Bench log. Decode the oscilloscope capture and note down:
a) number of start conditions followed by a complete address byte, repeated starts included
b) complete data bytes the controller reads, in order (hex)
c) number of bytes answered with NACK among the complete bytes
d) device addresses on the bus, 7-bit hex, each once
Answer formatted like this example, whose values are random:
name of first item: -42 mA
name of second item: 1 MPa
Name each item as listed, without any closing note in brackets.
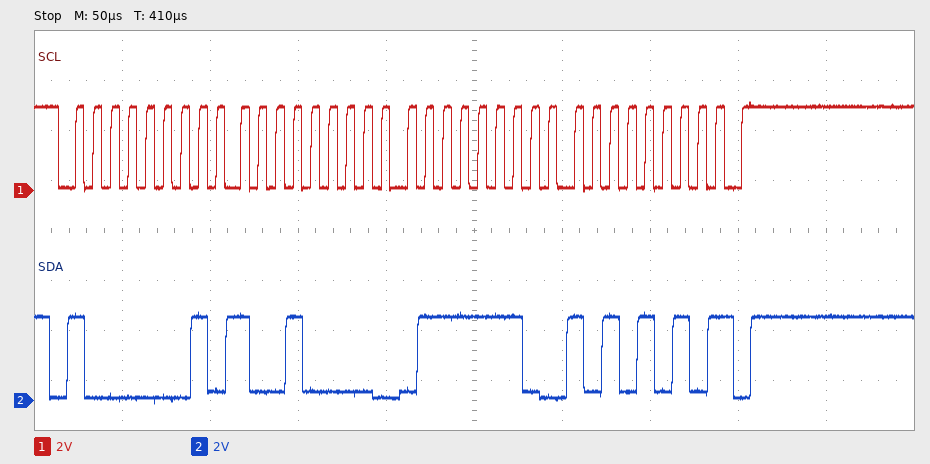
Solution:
number of start conditions followed by a complete address byte, repeated starts included: 1
complete data bytes the controller reads, in order: 90 7E AA
number of bytes answered with NACK among the complete bytes: 1
device addresses on the bus, 7-bit hex, each once: 0x40
